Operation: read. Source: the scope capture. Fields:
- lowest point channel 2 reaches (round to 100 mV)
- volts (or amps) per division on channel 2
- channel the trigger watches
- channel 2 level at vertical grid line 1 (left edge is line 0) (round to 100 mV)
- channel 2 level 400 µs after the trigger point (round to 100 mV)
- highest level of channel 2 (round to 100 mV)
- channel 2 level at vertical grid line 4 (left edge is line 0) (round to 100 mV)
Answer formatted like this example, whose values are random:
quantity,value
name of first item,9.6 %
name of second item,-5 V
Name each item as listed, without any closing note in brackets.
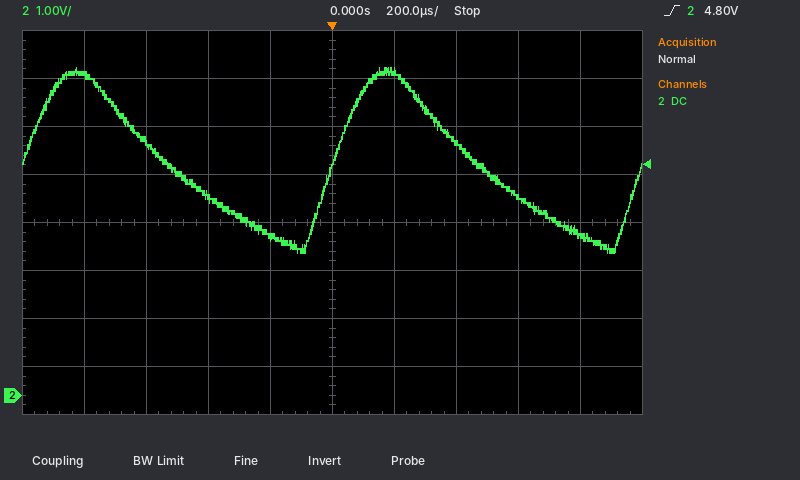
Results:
quantity,value
lowest point channel 2 reaches,3.0 V
volts (or amps) per division on channel 2,1 V
channel the trigger watches,channel 2
channel 2 level at vertical grid line 1 (left edge is line 0),6.7 V
channel 2 level 400 µs after the trigger point,5.3 V
highest level of channel 2,6.8 V
channel 2 level at vertical grid line 4 (left edge is line 0),3.3 V
